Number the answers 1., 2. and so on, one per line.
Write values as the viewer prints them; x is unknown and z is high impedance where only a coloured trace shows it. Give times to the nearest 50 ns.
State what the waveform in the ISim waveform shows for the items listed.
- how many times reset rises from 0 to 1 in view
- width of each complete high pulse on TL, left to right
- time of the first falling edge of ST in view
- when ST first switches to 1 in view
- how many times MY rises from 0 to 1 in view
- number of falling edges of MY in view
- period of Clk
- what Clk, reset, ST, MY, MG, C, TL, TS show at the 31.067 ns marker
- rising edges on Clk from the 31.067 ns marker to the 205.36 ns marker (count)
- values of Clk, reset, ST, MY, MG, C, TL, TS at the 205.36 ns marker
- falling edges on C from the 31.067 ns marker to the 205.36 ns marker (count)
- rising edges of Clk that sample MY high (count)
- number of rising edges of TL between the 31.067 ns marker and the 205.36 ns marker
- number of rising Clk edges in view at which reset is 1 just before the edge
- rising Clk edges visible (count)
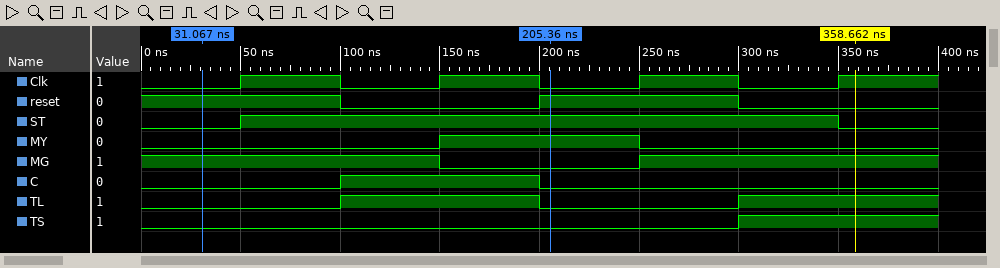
1. 1
2. 100 ns
3. 350 ns
4. 50 ns
5. 1
6. 1
7. 100 ns
8. Clk=0, reset=1, ST=0, MY=0, MG=1, C=0, TL=0, TS=0
9. 2
10. Clk=0, reset=1, ST=1, MY=1, MG=0, C=0, TL=0, TS=0
11. 1
12. 1
13. 1
14. 2
15. 4
